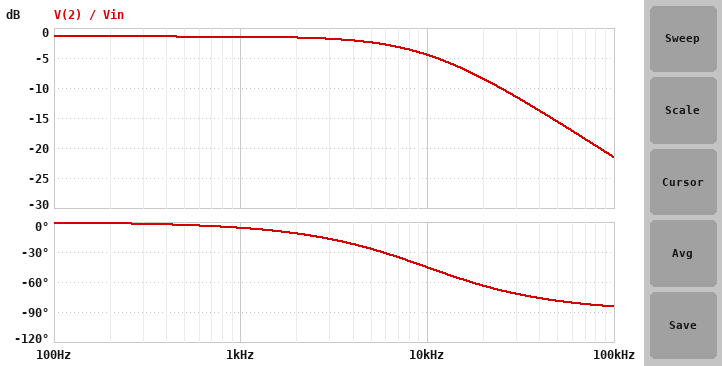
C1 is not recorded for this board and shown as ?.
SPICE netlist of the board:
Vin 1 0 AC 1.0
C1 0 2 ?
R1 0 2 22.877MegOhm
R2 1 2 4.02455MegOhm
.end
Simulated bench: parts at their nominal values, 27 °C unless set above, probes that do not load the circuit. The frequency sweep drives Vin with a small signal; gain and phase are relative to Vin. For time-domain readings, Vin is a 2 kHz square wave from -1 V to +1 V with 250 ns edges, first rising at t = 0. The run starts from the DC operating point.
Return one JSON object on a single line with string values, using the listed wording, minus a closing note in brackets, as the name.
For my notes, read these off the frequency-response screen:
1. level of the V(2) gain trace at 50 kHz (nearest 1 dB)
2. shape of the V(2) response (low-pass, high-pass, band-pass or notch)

{"level of the V(2) gain trace at 50 kHz": "-16 dB", "shape of the V(2) response": "low-pass"}
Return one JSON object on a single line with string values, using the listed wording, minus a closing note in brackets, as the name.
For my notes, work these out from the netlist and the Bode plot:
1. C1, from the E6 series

{"C1, from the E6 series": "4.7 pF"}
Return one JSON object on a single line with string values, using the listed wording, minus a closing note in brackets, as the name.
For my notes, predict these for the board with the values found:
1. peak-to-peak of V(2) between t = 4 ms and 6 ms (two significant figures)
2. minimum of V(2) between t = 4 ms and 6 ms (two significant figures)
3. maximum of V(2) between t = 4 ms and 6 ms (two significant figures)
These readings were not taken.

{"peak-to-peak of V(2) between t = 4 ms and 6 ms": "1.7 V", "minimum of V(2) between t = 4 ms and 6 ms": "-850 mV", "maximum of V(2) between t = 4 ms and 6 ms": "850 mV"}
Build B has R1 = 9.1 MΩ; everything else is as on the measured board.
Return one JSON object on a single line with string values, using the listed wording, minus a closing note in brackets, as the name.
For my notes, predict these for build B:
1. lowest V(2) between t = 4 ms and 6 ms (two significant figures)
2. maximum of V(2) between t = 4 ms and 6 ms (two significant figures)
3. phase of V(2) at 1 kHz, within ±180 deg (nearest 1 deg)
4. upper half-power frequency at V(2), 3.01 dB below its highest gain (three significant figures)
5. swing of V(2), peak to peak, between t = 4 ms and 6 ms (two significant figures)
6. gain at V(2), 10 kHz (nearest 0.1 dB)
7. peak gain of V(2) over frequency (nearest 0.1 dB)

{"lowest V(2) between t = 4 ms and 6 ms": "-690 mV", "maximum of V(2) between t = 4 ms and 6 ms": "690 mV", "phase of V(2) at 1 kHz, within ±180 deg": "-5 deg", "upper half-power frequency at V(2), 3.01 dB below its highest gain": "12.1 kHz", "swing of V(2), peak to peak, between t = 4 ms and 6 ms": "1.4 V", "gain at V(2), 10 kHz": "-5.4 dB", "peak gain of V(2) over frequency": "-3.2 dB"}
